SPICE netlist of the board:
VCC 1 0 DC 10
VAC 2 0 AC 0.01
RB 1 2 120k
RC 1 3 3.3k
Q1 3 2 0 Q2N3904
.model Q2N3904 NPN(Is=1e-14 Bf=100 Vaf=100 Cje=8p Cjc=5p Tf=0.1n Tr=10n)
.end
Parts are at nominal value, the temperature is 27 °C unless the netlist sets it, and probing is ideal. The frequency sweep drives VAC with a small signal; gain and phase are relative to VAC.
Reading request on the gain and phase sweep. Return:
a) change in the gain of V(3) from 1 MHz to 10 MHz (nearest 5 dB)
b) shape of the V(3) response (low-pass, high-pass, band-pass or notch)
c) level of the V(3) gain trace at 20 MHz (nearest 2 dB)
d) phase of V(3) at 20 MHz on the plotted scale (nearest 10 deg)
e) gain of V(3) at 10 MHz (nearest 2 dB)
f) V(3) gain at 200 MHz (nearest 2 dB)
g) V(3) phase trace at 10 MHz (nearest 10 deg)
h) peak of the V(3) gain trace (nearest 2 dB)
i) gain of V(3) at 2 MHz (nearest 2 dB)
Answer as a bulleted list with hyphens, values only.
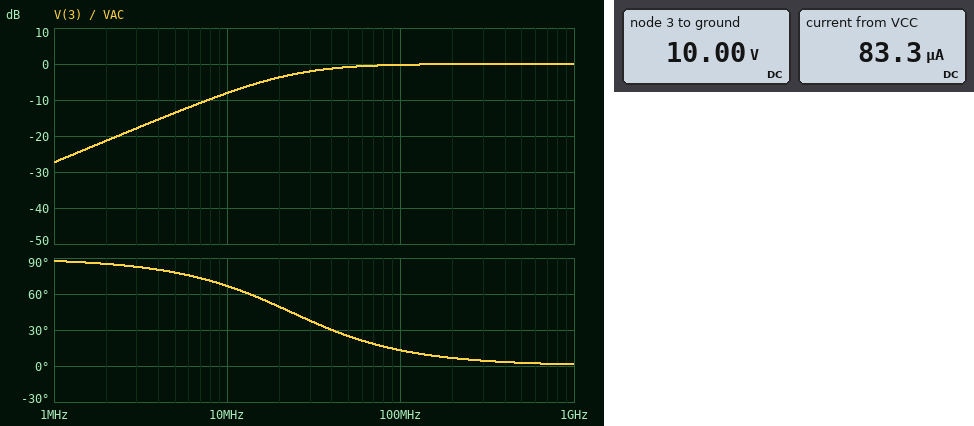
- 20 dB
- high-pass
- -4 dB
- 50 deg
- -8 dB
- 0 dB
- 70 deg
- 0 dB
- -22 dB
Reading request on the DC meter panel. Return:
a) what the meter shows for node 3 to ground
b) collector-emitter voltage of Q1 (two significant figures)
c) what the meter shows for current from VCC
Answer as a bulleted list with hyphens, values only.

- 10.00 V
- 10 V
- 83.3 µA
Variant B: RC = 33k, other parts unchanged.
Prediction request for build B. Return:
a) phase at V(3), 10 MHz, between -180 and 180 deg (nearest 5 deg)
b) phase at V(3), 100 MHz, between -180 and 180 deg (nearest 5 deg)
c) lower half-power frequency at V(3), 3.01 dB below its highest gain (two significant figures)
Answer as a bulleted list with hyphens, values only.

- 15 deg
- 0 deg
- 2.3 MHz
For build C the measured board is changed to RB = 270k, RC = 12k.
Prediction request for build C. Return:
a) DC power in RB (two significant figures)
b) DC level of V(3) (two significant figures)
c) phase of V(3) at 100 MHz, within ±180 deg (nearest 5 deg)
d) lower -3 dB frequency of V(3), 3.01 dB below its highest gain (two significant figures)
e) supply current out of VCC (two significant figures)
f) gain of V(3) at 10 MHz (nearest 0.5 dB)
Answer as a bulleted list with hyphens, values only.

- 370 µW
- 10 V
- 5 deg
- 6.4 MHz
- 37 µA
- -1.5 dB
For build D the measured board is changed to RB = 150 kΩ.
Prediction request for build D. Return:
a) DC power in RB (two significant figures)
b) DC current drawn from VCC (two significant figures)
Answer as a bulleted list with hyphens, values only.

- 670 µW
- 67 µA
